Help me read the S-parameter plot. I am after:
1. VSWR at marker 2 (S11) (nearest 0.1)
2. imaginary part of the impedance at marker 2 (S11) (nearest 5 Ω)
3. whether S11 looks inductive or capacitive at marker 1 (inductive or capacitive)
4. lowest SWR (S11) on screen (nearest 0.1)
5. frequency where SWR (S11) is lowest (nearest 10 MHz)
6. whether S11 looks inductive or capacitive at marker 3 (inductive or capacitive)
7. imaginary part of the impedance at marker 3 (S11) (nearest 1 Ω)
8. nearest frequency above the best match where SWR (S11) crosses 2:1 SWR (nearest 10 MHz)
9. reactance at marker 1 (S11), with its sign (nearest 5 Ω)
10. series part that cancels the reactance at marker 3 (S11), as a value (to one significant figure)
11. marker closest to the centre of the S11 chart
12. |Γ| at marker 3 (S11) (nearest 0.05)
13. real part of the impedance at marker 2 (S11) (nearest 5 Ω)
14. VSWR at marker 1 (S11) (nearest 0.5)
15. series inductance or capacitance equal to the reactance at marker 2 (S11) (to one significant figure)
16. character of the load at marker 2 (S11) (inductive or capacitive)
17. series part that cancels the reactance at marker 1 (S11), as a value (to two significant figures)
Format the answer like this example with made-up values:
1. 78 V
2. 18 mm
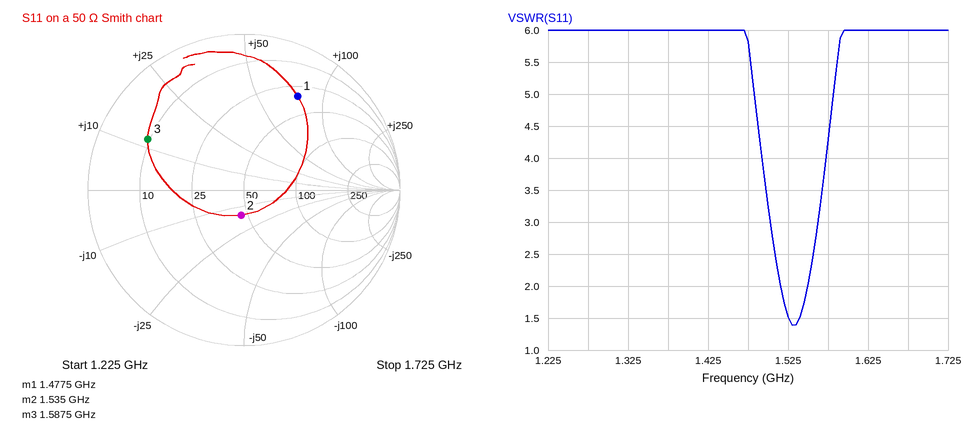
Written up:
1. 1.4
2. -15 Ω
3. inductive
4. 1.4
5. 1.53 GHz
6. inductive
7. +12 Ω
8. 1.55 GHz
9. +75 Ω
10. 8 pF
11. marker 2
12. 0.70
13. 45 Ω
14. 5.5
15. 7 pF
16. capacitive
17. 1.4 pF
